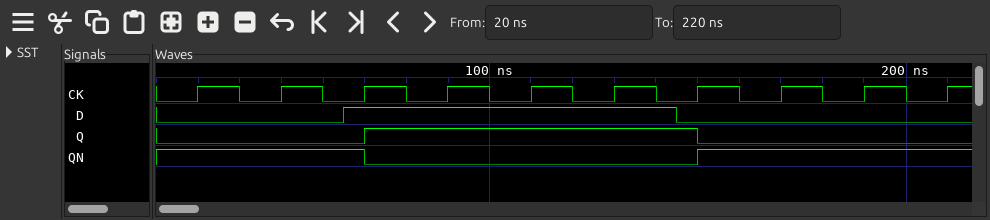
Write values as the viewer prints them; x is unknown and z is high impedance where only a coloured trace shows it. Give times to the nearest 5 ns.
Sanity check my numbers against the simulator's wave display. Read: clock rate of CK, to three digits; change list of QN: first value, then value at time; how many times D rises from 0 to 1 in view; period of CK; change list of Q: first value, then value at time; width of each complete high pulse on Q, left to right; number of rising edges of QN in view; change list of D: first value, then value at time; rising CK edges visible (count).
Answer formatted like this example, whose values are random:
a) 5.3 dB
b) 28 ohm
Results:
a) 50.0 MHz
b) 1, 0 at 70 ns, 1 at 150 ns
c) 1
d) 20 ns
e) 0, 1 at 70 ns, 0 at 150 ns
f) 80 ns
g) 1
h) 0, 1 at 65 ns, 0 at 145 ns
i) 10
